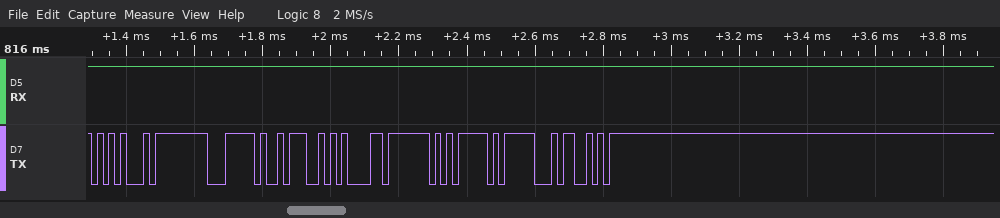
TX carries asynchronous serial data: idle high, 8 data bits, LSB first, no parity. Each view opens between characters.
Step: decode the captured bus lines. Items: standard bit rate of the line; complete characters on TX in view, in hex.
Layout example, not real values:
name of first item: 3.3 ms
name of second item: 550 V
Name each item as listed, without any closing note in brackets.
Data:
standard bit rate of the line: 57600 baud
complete characters on TX in view, in hex: 15, FF, 7C, 3A, 85, 7F, 7D, 1F, 53
